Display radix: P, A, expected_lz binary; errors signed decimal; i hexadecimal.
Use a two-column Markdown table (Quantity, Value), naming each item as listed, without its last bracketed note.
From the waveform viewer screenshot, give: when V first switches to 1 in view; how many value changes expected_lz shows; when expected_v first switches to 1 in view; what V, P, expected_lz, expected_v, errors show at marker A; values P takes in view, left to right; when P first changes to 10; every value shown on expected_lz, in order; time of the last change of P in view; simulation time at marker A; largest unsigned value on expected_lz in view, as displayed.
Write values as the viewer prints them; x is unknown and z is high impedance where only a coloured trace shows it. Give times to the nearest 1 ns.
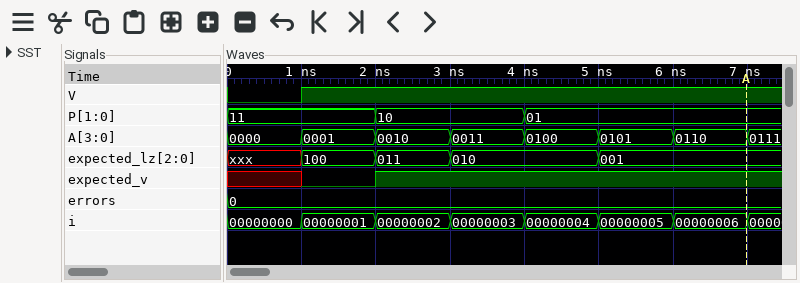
| Quantity | Value |
|---|---|
| when V first switches to 1 in view | 1 ns |
| how many value changes expected_lz shows | 4 |
| when expected_v first switches to 1 in view | 2 ns |
| what V, P, expected_lz, expected_v, errors show at marker A | V=1, P=01, expected_lz=001, expected_v=1, errors=0 |
| values P takes in view, left to right | 11, 10, 01 |
| when P first changes to 10 | 2 ns |
| every value shown on expected_lz, in order | xxx, 100, 011, 010, 001 |
| time of the last change of P in view | 4 ns |
| simulation time at marker A | 7 ns |
| largest unsigned value on expected_lz in view, as displayed | 100 |
